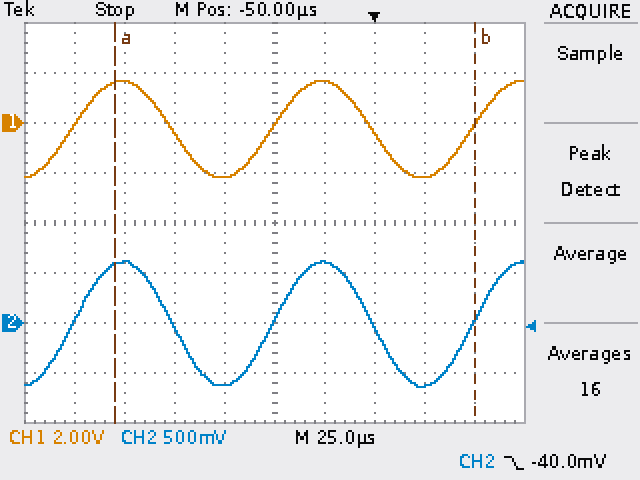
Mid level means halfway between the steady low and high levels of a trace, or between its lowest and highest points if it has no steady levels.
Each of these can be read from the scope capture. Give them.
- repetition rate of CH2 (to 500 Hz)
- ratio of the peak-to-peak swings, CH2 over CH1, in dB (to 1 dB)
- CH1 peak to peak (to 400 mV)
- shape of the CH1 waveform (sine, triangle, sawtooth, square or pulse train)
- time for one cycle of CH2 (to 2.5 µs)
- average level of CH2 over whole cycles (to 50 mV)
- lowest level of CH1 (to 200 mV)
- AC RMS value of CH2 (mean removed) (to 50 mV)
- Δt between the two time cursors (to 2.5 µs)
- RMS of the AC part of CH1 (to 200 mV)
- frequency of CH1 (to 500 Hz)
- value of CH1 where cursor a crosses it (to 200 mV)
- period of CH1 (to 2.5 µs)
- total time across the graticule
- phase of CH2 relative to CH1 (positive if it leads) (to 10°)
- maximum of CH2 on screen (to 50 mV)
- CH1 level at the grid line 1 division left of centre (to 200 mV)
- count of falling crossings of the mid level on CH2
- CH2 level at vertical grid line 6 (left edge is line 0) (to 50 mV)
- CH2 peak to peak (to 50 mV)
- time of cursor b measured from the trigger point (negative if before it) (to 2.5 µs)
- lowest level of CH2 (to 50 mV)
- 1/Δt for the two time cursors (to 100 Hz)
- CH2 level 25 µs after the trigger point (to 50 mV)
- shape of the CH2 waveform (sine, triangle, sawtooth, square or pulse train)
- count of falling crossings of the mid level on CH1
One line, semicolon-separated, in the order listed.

10.0 kHz; -10 dB; 4.0 V; sine; 100.0 µs; 0 mV; -2.2 V; 450 mV; 180.0 µs; 1.4 V; 10.0 kHz; 1.6 V; 100.0 µs; 250 µs; 0°; 600 mV; -2.2 V; 2; 600 mV; 1.25 V; +50.0 µs; -650 mV; 5.6 kHz; -650 mV; sine; 2
